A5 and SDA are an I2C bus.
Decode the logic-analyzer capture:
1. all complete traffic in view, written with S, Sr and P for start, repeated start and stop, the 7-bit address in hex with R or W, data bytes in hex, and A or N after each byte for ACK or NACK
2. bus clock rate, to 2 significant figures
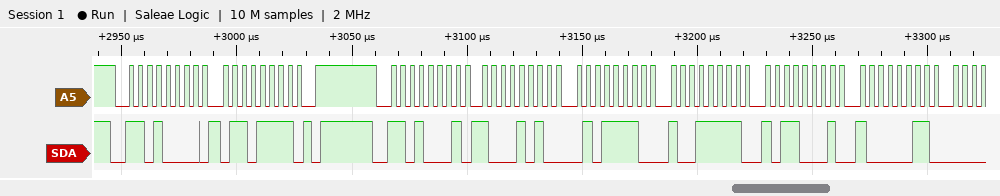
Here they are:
S 68W A 6F A P S 68R A 8A A 5E A 9F A B1 A 83 A
250 kHz
